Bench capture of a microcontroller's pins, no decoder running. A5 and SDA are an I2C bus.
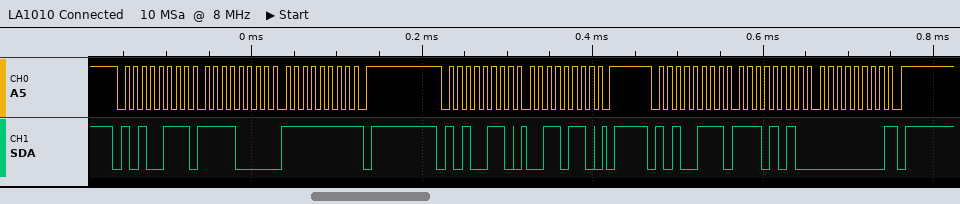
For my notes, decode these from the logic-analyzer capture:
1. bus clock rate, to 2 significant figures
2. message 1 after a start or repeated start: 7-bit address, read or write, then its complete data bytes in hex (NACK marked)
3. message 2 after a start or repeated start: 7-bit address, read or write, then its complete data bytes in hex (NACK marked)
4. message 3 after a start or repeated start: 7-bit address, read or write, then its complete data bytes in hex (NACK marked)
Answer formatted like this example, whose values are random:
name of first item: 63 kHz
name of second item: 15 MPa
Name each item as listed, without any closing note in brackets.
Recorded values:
bus clock rate, to 2 significant figures: 100 kHz
message 1 after a start or repeated start: 7-bit address, read or write, then its complete data bytes in hex: 0x53 read: F0 FF NACK
message 2 after a start or repeated start: 7-bit address, read or write, then its complete data bytes in hex: 0x53 write: 36
message 3 after a start or repeated start: 7-bit address, read or write, then its complete data bytes in hex: 0x53 read: EA 00 NACK
